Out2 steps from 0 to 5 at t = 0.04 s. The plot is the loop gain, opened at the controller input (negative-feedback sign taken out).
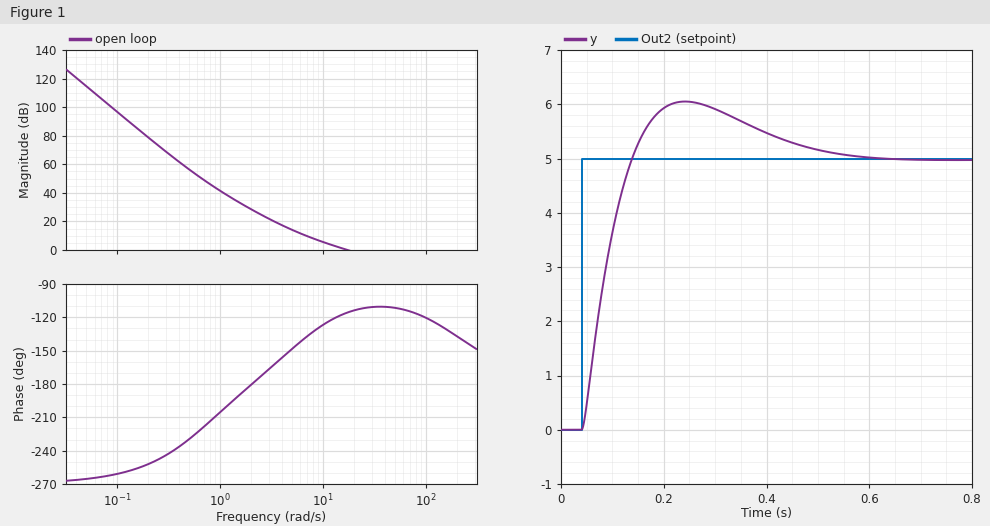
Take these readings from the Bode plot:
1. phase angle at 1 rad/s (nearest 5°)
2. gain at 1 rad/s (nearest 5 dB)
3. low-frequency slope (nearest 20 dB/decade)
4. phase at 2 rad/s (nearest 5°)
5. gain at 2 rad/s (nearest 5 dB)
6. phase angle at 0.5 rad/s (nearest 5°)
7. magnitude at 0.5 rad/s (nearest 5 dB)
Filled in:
-205°
40 dB
-60 dB/decade
-180°
30 dB
-230°
55 dB
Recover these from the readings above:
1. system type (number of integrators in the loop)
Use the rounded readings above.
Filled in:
3
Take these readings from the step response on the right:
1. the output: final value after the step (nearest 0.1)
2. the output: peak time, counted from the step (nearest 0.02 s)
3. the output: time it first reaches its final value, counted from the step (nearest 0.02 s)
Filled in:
5.0
0.20 s
0.10 s
